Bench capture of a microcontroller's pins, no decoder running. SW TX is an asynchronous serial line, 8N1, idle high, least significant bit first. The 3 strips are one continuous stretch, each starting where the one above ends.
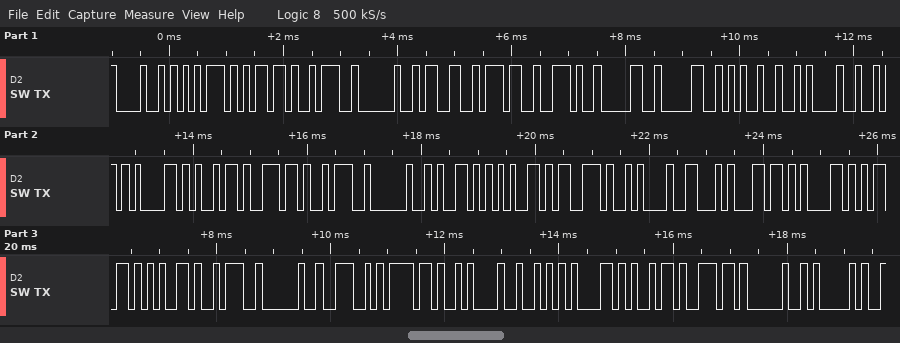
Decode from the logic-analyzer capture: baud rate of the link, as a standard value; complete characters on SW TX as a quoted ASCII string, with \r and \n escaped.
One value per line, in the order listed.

9600 baud
"Hum: 37.00%\nRain: Yes\nFlame: No\nRain A"
